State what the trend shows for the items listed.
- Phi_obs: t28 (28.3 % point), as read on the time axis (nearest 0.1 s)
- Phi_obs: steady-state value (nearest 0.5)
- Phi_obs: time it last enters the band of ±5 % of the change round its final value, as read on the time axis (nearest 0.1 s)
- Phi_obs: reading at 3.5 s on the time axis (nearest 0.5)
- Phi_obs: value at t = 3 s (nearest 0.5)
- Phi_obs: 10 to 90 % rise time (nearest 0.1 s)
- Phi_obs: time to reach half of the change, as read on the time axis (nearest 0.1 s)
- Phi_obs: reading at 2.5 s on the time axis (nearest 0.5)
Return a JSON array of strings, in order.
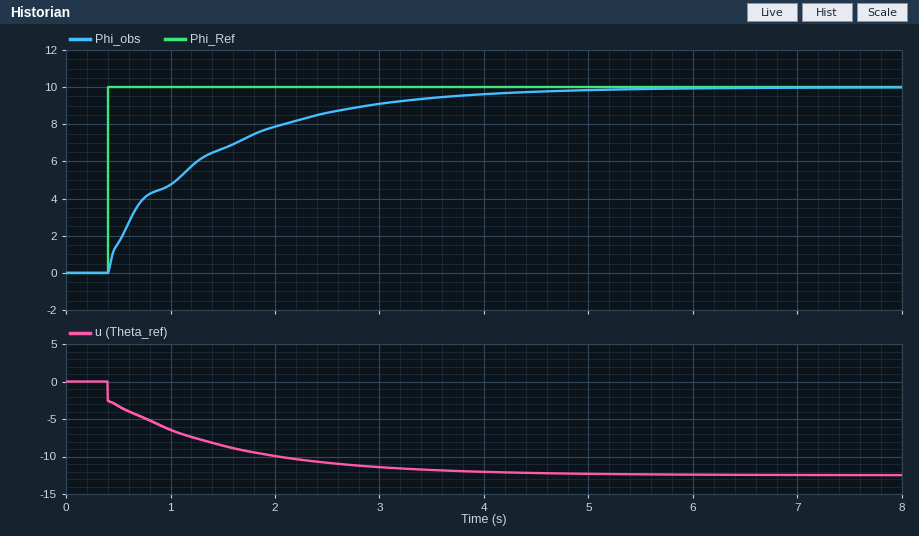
["0.6 s", "10.0", "3.7 s", "9.5", "9.0", "2.4 s", "1.1 s", "8.5"]
